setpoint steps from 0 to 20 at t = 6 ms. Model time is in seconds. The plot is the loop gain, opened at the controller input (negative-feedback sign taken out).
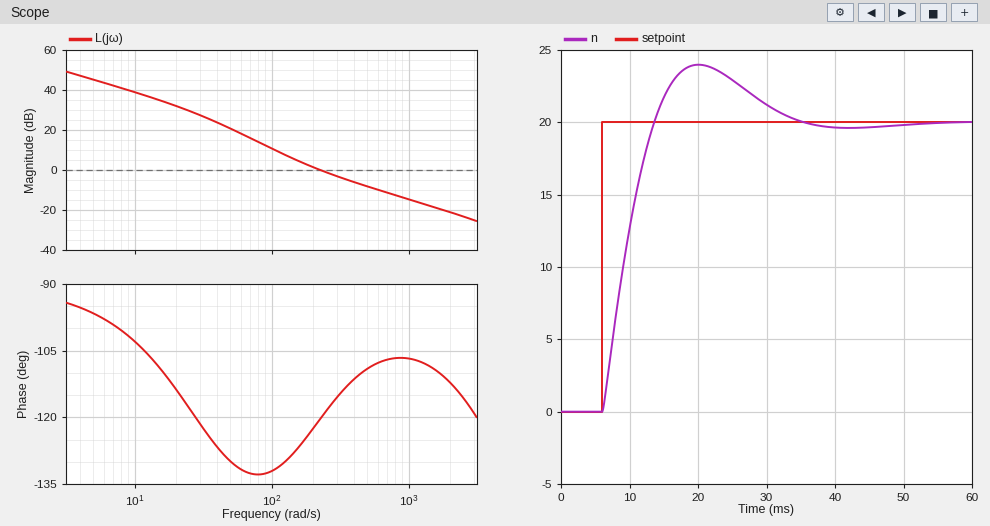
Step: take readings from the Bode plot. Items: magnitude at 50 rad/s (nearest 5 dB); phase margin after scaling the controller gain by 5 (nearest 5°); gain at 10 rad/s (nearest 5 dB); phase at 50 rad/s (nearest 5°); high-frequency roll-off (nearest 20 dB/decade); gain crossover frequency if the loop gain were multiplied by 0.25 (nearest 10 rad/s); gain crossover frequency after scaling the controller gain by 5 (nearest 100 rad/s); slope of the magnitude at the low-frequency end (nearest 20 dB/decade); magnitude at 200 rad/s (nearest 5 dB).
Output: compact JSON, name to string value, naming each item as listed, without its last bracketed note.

{"magnitude at 50 rad/s": "20 dB", "phase margin after scaling the controller gain by 5": "75°", "gain at 10 rad/s": "40 dB", "phase at 50 rad/s": "-130°", "high-frequency roll-off": "-20 dB/decade", "gain crossover frequency if the loop gain were multiplied by 0.25": "90 rad/s", "gain crossover frequency after scaling the controller gain by 5": "900 rad/s", "slope of the magnitude at the low-frequency end": "-20 dB/decade", "magnitude at 200 rad/s": "0 dB"}
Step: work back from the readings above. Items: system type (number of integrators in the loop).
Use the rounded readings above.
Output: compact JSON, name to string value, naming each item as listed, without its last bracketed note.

{"system type": "1"}
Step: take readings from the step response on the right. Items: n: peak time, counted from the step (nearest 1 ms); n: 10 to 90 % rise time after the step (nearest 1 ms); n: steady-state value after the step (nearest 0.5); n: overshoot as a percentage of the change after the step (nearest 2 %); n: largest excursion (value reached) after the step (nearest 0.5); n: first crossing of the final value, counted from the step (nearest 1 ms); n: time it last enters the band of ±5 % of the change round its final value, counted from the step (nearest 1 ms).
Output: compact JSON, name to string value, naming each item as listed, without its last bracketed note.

{"n: peak time, counted from the step": "14 ms", "n: 10 to 90 % rise time after the step": "6 ms", "n: steady-state value after the step": "20.0", "n: overshoot as a percentage of the change after the step": "20 %", "n: largest excursion (value reached) after the step": "24.0", "n: first crossing of the final value, counted from the step": "8 ms", "n: time it last enters the band of ±5 % of the change round its final value, counted from the step": "25 ms"}
